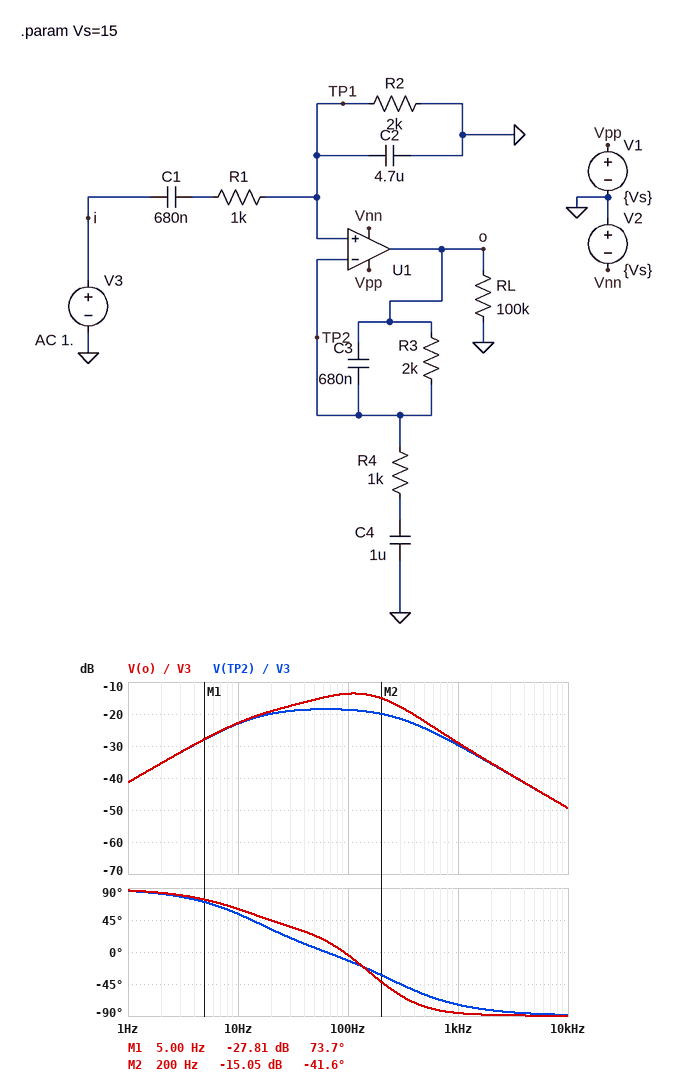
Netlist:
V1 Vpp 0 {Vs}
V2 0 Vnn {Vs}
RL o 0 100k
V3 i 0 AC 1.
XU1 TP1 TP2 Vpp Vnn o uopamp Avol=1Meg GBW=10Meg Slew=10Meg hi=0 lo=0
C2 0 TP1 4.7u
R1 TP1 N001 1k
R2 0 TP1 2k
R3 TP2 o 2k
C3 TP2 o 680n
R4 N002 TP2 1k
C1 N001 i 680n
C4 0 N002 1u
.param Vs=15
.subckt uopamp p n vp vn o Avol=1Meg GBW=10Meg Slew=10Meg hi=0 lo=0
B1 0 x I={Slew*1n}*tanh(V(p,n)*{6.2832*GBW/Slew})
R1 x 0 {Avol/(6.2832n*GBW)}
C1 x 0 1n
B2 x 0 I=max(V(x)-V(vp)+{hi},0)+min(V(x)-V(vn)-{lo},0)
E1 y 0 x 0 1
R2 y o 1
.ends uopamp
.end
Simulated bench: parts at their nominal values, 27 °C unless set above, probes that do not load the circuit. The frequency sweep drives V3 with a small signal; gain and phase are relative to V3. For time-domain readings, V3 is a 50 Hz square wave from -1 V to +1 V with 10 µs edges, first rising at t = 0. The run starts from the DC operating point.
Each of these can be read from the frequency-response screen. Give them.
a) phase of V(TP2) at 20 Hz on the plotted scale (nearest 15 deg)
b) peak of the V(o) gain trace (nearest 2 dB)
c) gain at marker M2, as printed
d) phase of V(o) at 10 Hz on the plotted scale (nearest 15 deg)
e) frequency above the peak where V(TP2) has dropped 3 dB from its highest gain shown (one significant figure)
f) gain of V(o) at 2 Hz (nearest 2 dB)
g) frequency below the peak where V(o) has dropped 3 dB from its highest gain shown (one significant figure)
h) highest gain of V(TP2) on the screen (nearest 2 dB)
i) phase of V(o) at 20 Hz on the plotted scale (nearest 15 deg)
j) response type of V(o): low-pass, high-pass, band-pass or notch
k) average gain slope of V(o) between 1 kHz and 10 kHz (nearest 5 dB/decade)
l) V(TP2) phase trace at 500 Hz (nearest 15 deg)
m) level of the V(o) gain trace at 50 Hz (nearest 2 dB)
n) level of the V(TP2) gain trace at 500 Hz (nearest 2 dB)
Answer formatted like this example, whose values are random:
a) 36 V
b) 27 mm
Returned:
a) 30 deg
b) -14 dB
c) -15.05 dB
d) 60 deg
e) 300 Hz
f) -36 dB
g) 40 Hz
h) -18 dB
i) 45 deg
j) band-pass
k) -20 dB/decade
l) -60 deg
m) -16 dB
n) -24 dB
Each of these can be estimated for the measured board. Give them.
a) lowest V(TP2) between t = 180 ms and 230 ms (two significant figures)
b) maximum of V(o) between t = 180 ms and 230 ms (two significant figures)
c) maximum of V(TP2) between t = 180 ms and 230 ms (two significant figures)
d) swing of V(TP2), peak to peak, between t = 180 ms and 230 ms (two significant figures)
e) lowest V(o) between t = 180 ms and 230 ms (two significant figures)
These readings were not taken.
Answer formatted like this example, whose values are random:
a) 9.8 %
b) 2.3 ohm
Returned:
a) -150 mV
b) 290 mV
c) 150 mV
d) 300 mV
e) -290 mV
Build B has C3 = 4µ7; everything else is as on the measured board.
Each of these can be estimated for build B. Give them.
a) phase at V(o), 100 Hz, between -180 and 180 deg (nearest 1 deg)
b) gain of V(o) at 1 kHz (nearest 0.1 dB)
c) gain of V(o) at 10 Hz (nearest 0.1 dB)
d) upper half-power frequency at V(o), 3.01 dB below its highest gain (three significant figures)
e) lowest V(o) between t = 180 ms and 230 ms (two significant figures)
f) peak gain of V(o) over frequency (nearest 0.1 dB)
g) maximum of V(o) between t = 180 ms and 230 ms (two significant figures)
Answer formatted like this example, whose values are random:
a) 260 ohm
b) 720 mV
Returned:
a) -15 deg
b) -29.7 dB
c) -22.5 dB
d) 242 Hz
e) -180 mV
f) -17.0 dB
g) 180 mV
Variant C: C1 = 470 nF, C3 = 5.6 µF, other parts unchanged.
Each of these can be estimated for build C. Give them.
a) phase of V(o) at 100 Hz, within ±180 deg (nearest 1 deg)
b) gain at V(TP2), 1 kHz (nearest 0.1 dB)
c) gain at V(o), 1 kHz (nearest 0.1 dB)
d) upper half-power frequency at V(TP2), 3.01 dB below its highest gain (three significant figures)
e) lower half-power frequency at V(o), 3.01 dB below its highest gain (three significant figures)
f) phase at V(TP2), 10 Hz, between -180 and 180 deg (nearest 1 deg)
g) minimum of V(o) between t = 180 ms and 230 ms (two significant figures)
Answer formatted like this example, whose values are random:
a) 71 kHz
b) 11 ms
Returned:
a) -9 deg
b) -30.0 dB
c) -29.9 dB
d) 404 Hz
e) 15.5 Hz
f) 55 deg
g) -130 mV
